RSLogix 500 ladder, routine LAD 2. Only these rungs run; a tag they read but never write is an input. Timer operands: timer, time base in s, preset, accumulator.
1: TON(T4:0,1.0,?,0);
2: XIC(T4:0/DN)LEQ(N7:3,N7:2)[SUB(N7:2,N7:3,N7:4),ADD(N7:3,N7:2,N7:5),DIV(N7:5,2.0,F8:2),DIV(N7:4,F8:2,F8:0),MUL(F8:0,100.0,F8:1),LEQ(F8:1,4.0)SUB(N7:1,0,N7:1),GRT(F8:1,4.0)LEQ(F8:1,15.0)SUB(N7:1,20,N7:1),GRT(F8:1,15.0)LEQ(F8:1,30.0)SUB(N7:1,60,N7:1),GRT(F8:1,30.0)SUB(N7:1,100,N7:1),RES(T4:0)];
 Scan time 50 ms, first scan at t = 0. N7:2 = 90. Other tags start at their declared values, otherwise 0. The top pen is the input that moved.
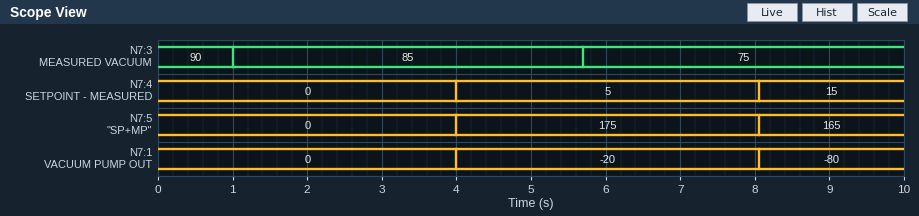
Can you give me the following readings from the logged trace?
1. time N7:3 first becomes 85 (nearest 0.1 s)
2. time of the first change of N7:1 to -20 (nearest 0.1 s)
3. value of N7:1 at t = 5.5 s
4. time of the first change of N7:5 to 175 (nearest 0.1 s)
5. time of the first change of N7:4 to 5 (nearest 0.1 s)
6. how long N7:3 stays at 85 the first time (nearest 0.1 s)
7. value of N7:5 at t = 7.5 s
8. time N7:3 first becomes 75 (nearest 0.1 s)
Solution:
1.0 s
4.0 s
-20
4.0 s
4.0 s
4.7 s
175
5.7 s
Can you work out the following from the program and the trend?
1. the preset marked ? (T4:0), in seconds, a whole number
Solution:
4 s
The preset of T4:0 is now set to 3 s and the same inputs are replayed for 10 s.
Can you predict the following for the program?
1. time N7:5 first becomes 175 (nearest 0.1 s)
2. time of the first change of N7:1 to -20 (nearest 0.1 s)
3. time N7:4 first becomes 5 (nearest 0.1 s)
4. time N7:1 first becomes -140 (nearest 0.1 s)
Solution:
3.0 s
3.0 s
3.0 s
9.1 s
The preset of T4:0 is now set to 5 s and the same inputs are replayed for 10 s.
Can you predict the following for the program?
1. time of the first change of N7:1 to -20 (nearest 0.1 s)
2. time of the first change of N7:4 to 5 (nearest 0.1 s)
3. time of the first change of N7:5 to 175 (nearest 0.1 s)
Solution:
5.0 s
5.0 s
5.0 s
